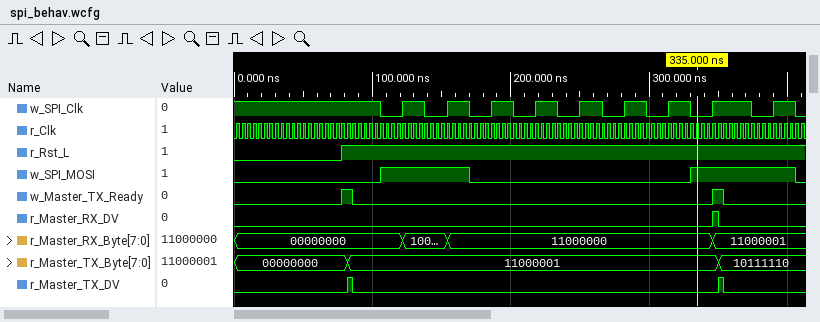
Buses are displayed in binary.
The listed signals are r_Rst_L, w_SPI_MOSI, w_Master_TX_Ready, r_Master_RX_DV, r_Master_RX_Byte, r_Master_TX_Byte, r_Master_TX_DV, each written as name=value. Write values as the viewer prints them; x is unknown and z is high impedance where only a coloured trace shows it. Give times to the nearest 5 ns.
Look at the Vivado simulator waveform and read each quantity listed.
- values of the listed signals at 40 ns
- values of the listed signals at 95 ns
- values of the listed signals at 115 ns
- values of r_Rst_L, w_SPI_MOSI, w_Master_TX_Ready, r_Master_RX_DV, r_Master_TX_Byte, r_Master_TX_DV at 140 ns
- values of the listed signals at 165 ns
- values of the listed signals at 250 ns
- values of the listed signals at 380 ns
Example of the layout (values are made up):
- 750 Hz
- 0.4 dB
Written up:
- r_Rst_L=0, w_SPI_MOSI=0, w_Master_TX_Ready=0, r_Master_RX_DV=0, r_Master_RX_Byte=00000000, r_Master_TX_Byte=00000000, r_Master_TX_DV=0
- r_Rst_L=1, w_SPI_MOSI=0, w_Master_TX_Ready=0, r_Master_RX_DV=0, r_Master_RX_Byte=00000000, r_Master_TX_Byte=11000001, r_Master_TX_DV=0
- r_Rst_L=1, w_SPI_MOSI=1, w_Master_TX_Ready=0, r_Master_RX_DV=0, r_Master_RX_Byte=00000000, r_Master_TX_Byte=11000001, r_Master_TX_DV=0
- r_Rst_L=1, w_SPI_MOSI=1, w_Master_TX_Ready=0, r_Master_RX_DV=0, r_Master_TX_Byte=11000001, r_Master_TX_DV=0
- r_Rst_L=1, w_SPI_MOSI=1, w_Master_TX_Ready=0, r_Master_RX_DV=0, r_Master_RX_Byte=11000000, r_Master_TX_Byte=11000001, r_Master_TX_DV=0
- r_Rst_L=1, w_SPI_MOSI=0, w_Master_TX_Ready=0, r_Master_RX_DV=0, r_Master_RX_Byte=11000000, r_Master_TX_Byte=11000001, r_Master_TX_DV=0
- r_Rst_L=1, w_SPI_MOSI=1, w_Master_TX_Ready=0, r_Master_RX_DV=0, r_Master_RX_Byte=11000001, r_Master_TX_Byte=10111110, r_Master_TX_DV=0
